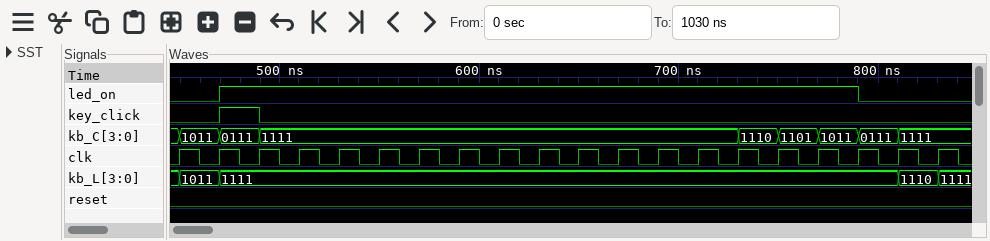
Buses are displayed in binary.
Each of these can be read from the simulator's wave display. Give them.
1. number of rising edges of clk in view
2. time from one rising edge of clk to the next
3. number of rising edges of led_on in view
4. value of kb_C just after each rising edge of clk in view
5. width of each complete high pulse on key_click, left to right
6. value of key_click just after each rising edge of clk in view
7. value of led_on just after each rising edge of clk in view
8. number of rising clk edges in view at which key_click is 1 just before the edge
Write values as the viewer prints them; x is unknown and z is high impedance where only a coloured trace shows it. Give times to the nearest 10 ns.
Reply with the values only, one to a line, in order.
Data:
20
20 ns
1
1011, 0111, 1111, 1111, 1111, 1111, 1111, 1111, 1111, 1111, 1111, 1111, 1111, 1111, 1110, 1101, 1011, 0111, 1111, 1111
20 ns
0 1 0 0 0 0 0 0 0 0 0 0 0 0 0 0 0 0 0 0
0 1 1 1 1 1 1 1 1 1 1 1 1 1 1 1 1 0 0 0
1
